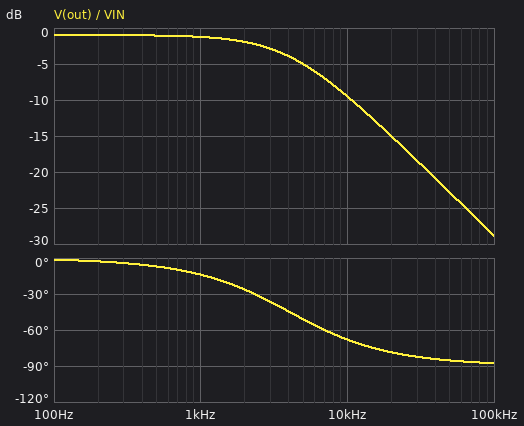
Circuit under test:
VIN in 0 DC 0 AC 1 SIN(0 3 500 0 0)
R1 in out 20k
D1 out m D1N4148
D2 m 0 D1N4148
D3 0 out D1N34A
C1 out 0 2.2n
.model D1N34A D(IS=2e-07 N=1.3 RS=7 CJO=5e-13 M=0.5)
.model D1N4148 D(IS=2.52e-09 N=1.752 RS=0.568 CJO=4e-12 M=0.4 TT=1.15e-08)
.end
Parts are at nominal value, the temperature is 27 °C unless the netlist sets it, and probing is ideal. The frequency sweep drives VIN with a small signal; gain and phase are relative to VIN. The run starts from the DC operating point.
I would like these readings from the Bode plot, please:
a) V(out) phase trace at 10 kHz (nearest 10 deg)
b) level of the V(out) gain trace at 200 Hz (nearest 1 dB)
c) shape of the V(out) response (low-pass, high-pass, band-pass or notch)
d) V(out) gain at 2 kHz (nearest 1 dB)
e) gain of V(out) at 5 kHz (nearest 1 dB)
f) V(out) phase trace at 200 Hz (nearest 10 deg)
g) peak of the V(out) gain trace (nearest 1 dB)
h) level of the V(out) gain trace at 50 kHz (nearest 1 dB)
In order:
-70 deg
-1 dB
low-pass
-2 dB
-5 dB
0 deg
-1 dB
-23 dB
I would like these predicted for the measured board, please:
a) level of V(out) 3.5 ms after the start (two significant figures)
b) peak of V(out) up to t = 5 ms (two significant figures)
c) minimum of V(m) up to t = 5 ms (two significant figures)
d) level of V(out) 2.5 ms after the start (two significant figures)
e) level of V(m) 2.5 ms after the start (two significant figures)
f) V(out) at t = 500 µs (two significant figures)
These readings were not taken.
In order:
-220 mV
960 mV
-110 mV
960 mV
480 mV
960 mV
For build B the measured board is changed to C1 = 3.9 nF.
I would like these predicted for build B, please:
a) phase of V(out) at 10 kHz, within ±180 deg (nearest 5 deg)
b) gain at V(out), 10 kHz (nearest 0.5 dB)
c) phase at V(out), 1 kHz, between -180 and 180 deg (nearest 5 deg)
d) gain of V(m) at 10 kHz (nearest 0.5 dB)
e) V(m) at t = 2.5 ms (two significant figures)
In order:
-75 deg
-14.0 dB
-25 deg
-20.0 dB
480 mV
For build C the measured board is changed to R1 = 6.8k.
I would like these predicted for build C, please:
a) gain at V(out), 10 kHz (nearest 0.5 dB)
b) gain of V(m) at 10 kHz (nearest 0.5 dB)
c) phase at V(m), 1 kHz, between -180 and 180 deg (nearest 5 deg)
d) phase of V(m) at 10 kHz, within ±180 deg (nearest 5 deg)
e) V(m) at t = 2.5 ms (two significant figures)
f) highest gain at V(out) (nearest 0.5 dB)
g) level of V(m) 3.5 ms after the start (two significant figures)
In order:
-3.0 dB
-9.0 dB
-5 deg
-40 deg
530 mV
-0.5 dB
-130 mV
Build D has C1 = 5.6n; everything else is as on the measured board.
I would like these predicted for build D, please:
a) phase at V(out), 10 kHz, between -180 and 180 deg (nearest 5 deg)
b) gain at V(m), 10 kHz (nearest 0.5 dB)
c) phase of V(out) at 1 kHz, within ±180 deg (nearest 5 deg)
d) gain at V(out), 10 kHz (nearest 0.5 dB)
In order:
-80 deg
-23.0 dB
-30 deg
-17.0 dB
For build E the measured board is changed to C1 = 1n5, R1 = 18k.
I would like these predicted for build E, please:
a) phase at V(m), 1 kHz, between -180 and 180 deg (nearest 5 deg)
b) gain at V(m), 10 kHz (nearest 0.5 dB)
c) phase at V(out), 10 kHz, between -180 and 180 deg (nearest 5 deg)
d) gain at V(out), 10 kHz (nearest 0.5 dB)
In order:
-10 deg
-12.0 dB
-55 deg
-6.0 dB
